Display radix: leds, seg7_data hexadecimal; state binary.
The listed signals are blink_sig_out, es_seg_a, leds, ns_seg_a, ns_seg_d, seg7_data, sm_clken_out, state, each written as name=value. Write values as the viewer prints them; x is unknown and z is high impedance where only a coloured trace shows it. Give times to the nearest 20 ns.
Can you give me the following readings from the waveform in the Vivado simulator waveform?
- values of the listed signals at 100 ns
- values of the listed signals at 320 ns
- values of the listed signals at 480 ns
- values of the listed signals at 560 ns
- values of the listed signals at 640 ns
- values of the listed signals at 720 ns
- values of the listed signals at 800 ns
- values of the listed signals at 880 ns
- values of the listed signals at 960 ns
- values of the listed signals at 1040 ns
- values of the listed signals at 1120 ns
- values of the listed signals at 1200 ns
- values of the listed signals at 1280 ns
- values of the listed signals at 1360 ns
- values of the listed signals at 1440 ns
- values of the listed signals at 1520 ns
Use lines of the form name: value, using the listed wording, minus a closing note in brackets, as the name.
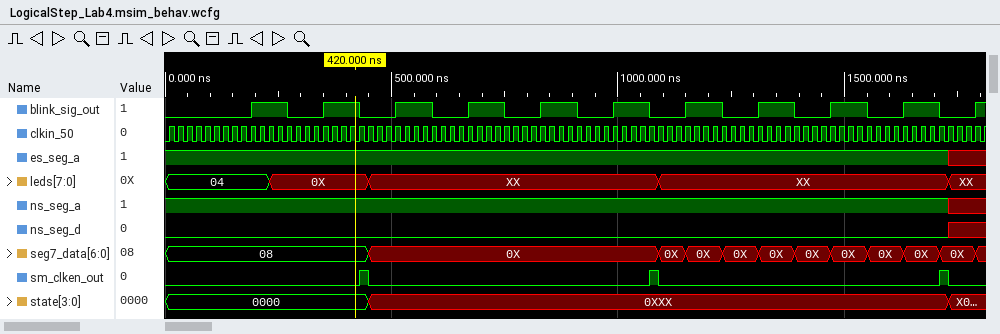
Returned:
values of the listed signals at 100 ns: blink_sig_out=0, es_seg_a=1, leds=04, ns_seg_a=1, ns_seg_d=0, seg7_data=08, sm_clken_out=0, state=0000
values of the listed signals at 320 ns: blink_sig_out=0, es_seg_a=1, leds=0X, ns_seg_a=1, ns_seg_d=0, seg7_data=08, sm_clken_out=0, state=0000
values of the listed signals at 480 ns: blink_sig_out=0, es_seg_a=1, leds=XX, ns_seg_a=1, ns_seg_d=0, seg7_data=0X, sm_clken_out=0, state=0XXX
values of the listed signals at 560 ns: blink_sig_out=1, es_seg_a=1, leds=XX, ns_seg_a=1, ns_seg_d=0, seg7_data=0X, sm_clken_out=0, state=0XXX
values of the listed signals at 640 ns: blink_sig_out=0, es_seg_a=1, leds=XX, ns_seg_a=1, ns_seg_d=0, seg7_data=0X, sm_clken_out=0, state=0XXX
values of the listed signals at 720 ns: blink_sig_out=1, es_seg_a=1, leds=XX, ns_seg_a=1, ns_seg_d=0, seg7_data=0X, sm_clken_out=0, state=0XXX
values of the listed signals at 800 ns: blink_sig_out=0, es_seg_a=1, leds=XX, ns_seg_a=1, ns_seg_d=0, seg7_data=0X, sm_clken_out=0, state=0XXX
values of the listed signals at 880 ns: blink_sig_out=1, es_seg_a=1, leds=XX, ns_seg_a=1, ns_seg_d=0, seg7_data=0X, sm_clken_out=0, state=0XXX
values of the listed signals at 960 ns: blink_sig_out=0, es_seg_a=1, leds=XX, ns_seg_a=1, ns_seg_d=0, seg7_data=0X, sm_clken_out=0, state=0XXX
values of the listed signals at 1040 ns: blink_sig_out=1, es_seg_a=1, leds=XX, ns_seg_a=1, ns_seg_d=0, seg7_data=0X, sm_clken_out=0, state=0XXX
values of the listed signals at 1120 ns: blink_sig_out=0, es_seg_a=1, leds=XX, ns_seg_a=1, ns_seg_d=0, seg7_data=0X, sm_clken_out=0, state=0XXX
values of the listed signals at 1200 ns: blink_sig_out=1, es_seg_a=1, leds=XX, ns_seg_a=1, ns_seg_d=0, seg7_data=0X, sm_clken_out=0, state=0XXX
values of the listed signals at 1280 ns: blink_sig_out=0, es_seg_a=1, leds=XX, ns_seg_a=1, ns_seg_d=0, seg7_data=0X, sm_clken_out=0, state=0XXX
values of the listed signals at 1360 ns: blink_sig_out=1, es_seg_a=1, leds=XX, ns_seg_a=1, ns_seg_d=0, seg7_data=0X, sm_clken_out=0, state=0XXX
values of the listed signals at 1440 ns: blink_sig_out=0, es_seg_a=1, leds=XX, ns_seg_a=1, ns_seg_d=0, seg7_data=0X, sm_clken_out=0, state=0XXX
values of the listed signals at 1520 ns: blink_sig_out=1, es_seg_a=1, leds=XX, ns_seg_a=1, ns_seg_d=0, seg7_data=0X, sm_clken_out=0, state=0XXX
